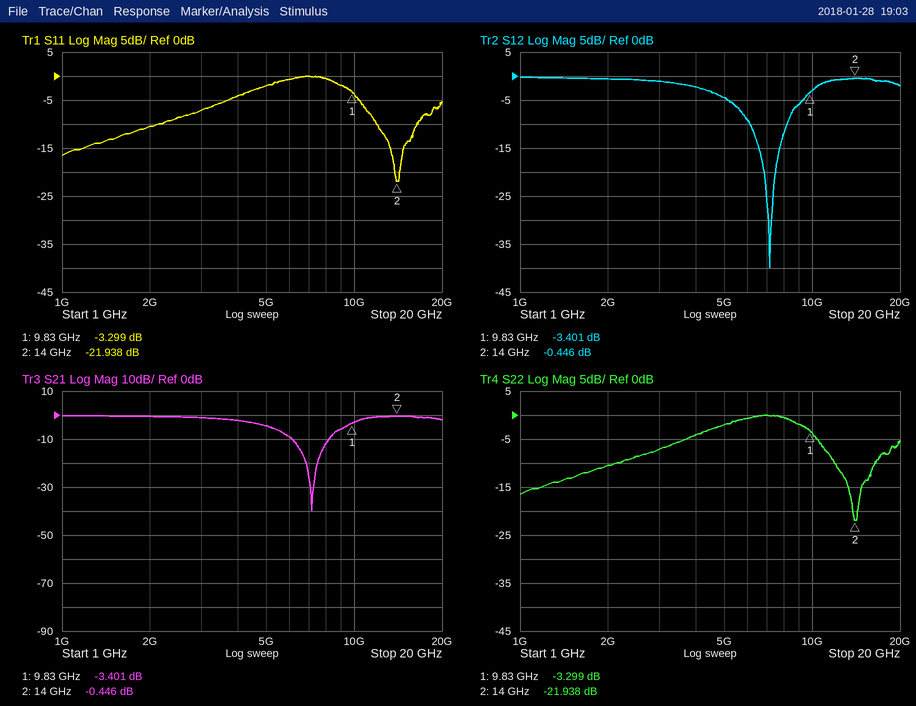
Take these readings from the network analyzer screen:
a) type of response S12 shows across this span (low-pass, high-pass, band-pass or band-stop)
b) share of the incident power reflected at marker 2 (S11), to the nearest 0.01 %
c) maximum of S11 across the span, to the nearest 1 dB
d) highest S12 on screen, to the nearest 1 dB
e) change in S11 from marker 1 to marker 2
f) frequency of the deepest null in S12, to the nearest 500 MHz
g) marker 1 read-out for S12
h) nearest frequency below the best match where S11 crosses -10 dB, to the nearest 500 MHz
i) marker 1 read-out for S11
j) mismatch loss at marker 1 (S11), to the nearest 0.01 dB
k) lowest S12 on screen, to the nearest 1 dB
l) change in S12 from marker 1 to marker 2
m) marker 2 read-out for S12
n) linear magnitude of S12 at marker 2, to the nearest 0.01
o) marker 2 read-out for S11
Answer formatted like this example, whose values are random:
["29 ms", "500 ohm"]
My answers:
["band-stop", "0.64 %", "0 dB", "0 dB", "-18.639 dB", "7.0 GHz", "-3.401 dB", "12.0 GHz", "-3.299 dB", "2.74 dB", "-40 dB", "2.955 dB", "-0.446 dB", "0.95", "-21.938 dB"]
